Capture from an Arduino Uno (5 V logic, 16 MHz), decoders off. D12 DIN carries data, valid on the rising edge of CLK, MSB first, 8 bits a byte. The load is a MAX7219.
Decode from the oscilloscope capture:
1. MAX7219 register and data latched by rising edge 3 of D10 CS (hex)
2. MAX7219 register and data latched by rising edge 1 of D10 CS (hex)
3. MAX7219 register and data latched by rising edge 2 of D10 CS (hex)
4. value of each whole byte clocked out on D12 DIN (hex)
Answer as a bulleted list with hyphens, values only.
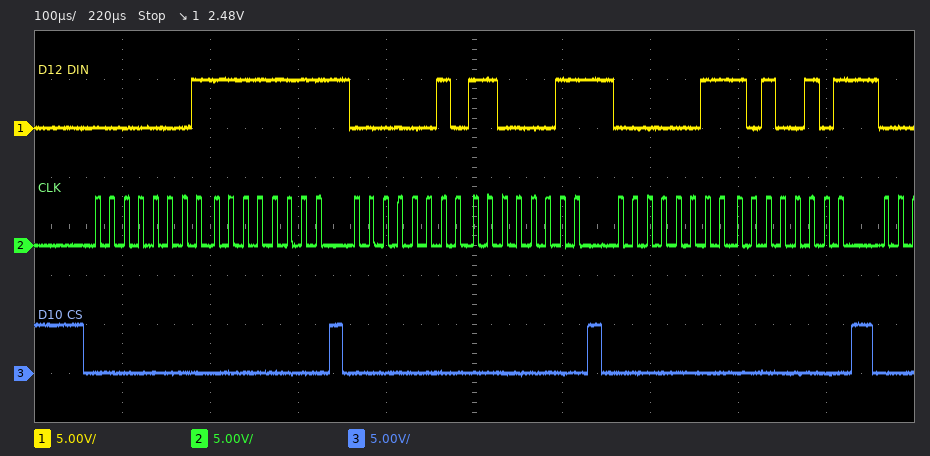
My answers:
- register 0x3, data 0xA5
- register 0x1, data 0xFF
- register 0x2, data 0xC3
- 01 FF 02 C3 03 A5
